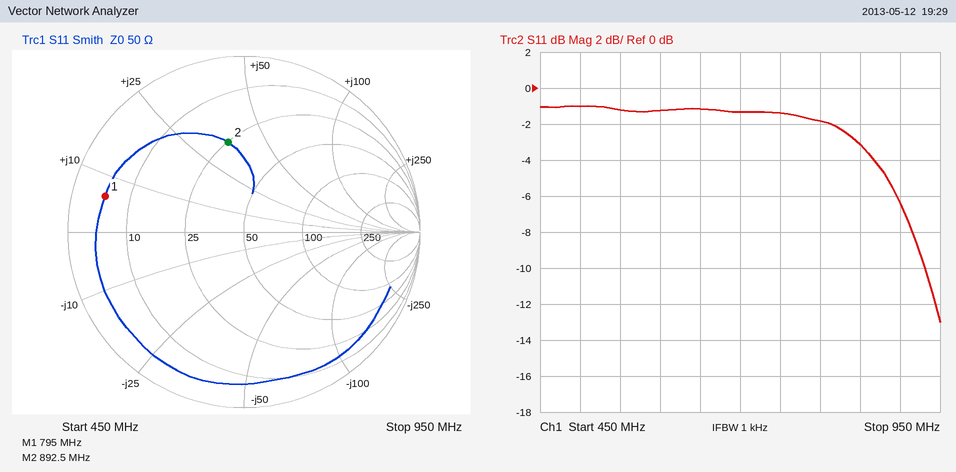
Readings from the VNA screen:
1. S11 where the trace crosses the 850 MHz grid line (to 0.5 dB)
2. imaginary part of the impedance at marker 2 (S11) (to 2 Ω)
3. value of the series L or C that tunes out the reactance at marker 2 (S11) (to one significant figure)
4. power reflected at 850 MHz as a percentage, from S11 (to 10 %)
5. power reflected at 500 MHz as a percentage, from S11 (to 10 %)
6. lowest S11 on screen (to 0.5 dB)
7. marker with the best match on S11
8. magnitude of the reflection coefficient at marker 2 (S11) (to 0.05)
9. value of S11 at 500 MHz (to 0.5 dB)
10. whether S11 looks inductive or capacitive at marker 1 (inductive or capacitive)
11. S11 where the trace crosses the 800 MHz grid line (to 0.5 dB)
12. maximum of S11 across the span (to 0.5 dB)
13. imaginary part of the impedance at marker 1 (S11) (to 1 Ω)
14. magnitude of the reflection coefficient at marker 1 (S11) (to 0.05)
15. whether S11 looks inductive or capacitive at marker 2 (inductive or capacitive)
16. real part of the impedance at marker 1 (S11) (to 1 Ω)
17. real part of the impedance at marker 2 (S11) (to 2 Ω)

-3.0 dB
+36 Ω
5 pF
50 %
80 %
-13.0 dB
marker 2
0.50
-1.0 dB
inductive
-2.0 dB
-1.0 dB
+6 Ω
0.80
inductive
5 Ω
26 Ω
